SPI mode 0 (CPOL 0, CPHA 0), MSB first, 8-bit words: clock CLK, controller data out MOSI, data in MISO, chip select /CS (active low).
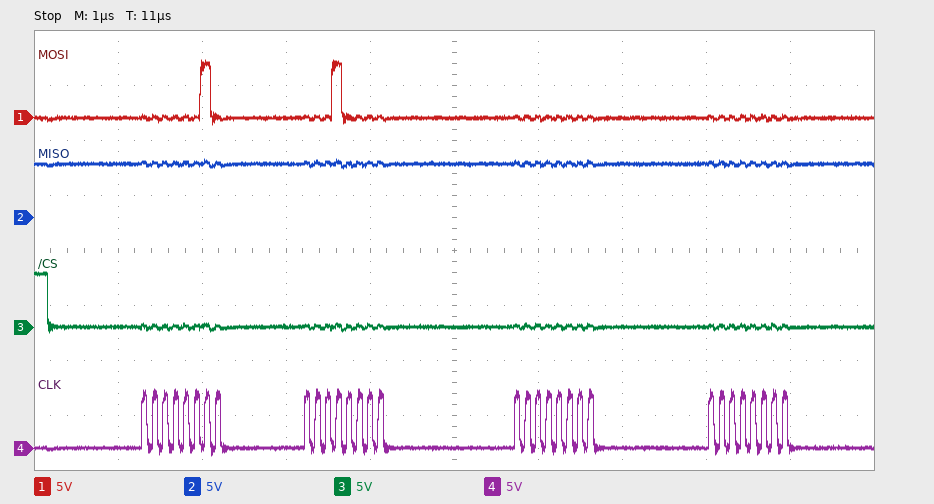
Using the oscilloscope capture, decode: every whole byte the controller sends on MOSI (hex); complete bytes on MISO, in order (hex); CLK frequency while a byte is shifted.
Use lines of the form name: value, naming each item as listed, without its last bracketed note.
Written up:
every whole byte the controller sends on MOSI: 02 10 00 00
complete bytes on MISO, in order: FF FF FF FF
CLK frequency while a byte is shifted: 8 MHz
